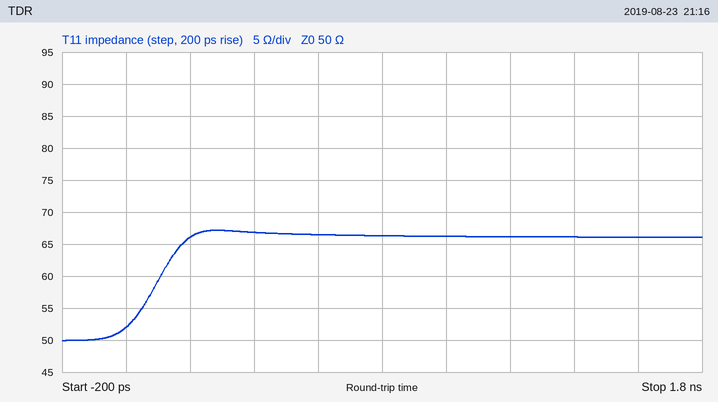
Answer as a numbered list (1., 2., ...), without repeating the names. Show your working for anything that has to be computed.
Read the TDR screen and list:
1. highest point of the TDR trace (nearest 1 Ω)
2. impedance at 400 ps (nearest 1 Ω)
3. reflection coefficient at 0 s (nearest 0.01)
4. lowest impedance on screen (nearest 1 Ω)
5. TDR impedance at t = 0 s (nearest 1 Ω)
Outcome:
1. 67 Ω
2. 67 Ω
3. (52 − 50)/(52 + 50) ≈ +0.02
4. 50 Ω
5. 52 Ω
